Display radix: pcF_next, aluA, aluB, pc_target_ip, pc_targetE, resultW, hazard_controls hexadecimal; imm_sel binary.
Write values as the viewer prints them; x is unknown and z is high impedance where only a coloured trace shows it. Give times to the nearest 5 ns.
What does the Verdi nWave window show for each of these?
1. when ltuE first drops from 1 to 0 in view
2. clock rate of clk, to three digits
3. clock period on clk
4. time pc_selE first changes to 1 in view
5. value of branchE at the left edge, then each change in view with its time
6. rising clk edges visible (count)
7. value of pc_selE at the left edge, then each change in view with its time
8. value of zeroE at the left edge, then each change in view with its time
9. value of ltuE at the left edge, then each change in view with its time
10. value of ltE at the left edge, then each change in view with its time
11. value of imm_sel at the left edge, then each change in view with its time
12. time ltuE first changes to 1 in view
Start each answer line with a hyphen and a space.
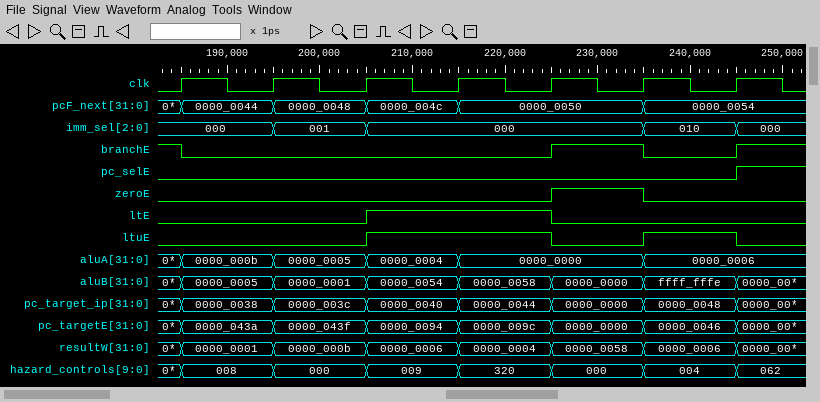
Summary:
- 225 ns
- 100 MHz
- 10 ns
- 245 ns
- 1, 0 at 185 ns, 1 at 225 ns, 0 at 235 ns, 1 at 245 ns
- 7
- 0, 1 at 245 ns
- 0, 1 at 225 ns, 0 at 235 ns
- 0, 1 at 205 ns, 0 at 225 ns, 1 at 235 ns, 0 at 245 ns
- 0, 1 at 205 ns, 0 at 225 ns
- 000, 001 at 195 ns, 000 at 205 ns, 010 at 235 ns, 000 at 245 ns
- 205 ns
